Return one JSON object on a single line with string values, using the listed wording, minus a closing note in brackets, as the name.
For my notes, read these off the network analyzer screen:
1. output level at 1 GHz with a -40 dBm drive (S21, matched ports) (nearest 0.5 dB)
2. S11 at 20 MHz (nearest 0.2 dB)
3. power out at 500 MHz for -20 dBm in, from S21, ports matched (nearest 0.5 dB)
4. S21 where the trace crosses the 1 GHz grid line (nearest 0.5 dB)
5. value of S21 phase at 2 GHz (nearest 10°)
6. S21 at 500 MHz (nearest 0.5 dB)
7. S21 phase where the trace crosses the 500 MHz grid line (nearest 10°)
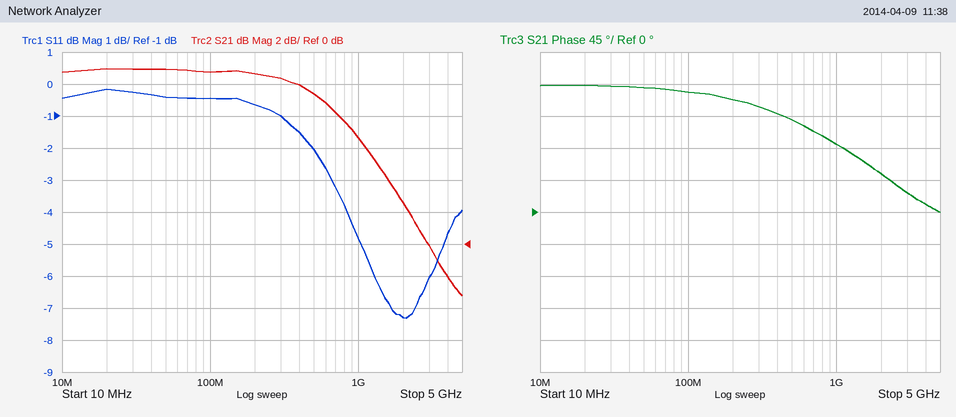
{"output level at 1 GHz with a -40 dBm drive (S21, matched ports)": "-33.5 dBm", "S11 at 20 MHz": "-0.2 dB", "power out at 500 MHz for -20 dBm in, from S21, ports matched": "-10.5 dBm", "S21 where the trace crosses the 1 GHz grid line": "6.5 dB", "value of S21 phase at 2 GHz": "50°", "S21 at 500 MHz": "9.5 dB", "S21 phase where the trace crosses the 500 MHz grid line": "130°"}
